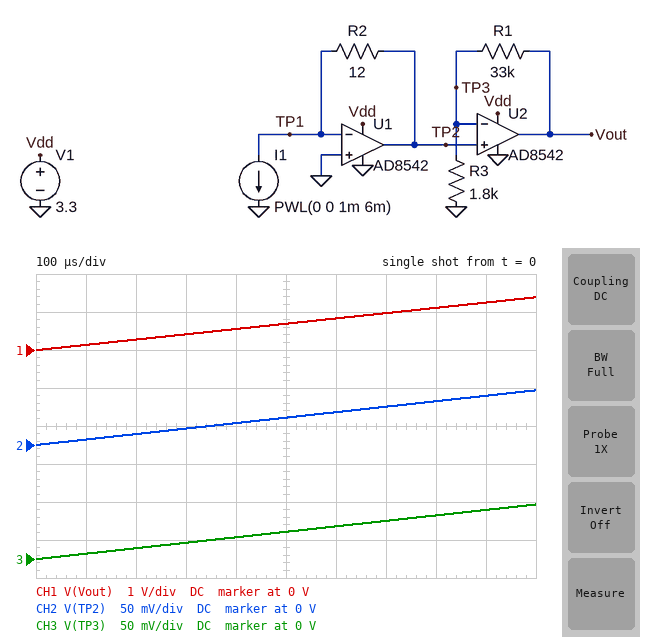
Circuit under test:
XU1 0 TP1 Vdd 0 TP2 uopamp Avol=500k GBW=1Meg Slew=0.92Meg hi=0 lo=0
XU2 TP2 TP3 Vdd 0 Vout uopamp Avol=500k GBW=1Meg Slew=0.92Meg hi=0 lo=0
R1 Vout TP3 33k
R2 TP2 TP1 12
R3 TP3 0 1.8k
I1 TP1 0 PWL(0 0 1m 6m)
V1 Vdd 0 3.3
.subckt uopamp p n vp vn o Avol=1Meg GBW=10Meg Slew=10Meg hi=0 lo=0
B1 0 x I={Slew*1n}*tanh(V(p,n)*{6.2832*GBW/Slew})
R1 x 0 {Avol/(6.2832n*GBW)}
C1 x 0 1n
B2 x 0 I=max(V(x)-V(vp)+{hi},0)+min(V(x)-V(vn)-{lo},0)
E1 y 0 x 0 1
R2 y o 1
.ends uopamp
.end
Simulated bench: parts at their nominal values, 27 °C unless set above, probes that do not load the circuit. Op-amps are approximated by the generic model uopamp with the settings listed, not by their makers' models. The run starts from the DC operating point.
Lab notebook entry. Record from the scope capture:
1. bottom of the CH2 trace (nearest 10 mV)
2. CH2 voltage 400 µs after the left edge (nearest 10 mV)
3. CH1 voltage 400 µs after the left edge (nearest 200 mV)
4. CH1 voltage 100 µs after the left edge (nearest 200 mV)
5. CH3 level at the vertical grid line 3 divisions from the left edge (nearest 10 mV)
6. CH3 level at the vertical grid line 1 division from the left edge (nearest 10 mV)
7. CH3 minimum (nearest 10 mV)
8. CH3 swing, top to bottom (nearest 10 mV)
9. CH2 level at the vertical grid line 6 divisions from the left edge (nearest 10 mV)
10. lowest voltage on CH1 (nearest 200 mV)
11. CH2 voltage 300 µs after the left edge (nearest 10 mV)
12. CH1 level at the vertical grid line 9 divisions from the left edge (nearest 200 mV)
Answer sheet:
0 V
30 mV
600 mV
200 mV
20 mV
10 mV
0 V
70 mV
40 mV
0 V
20 mV
1.2 V
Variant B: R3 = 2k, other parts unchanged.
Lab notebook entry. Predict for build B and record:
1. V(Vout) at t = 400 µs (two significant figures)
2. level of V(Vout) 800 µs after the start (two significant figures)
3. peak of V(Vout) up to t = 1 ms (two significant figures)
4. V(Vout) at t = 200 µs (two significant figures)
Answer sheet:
500 mV
1.0 V
1.3 V
250 mV
